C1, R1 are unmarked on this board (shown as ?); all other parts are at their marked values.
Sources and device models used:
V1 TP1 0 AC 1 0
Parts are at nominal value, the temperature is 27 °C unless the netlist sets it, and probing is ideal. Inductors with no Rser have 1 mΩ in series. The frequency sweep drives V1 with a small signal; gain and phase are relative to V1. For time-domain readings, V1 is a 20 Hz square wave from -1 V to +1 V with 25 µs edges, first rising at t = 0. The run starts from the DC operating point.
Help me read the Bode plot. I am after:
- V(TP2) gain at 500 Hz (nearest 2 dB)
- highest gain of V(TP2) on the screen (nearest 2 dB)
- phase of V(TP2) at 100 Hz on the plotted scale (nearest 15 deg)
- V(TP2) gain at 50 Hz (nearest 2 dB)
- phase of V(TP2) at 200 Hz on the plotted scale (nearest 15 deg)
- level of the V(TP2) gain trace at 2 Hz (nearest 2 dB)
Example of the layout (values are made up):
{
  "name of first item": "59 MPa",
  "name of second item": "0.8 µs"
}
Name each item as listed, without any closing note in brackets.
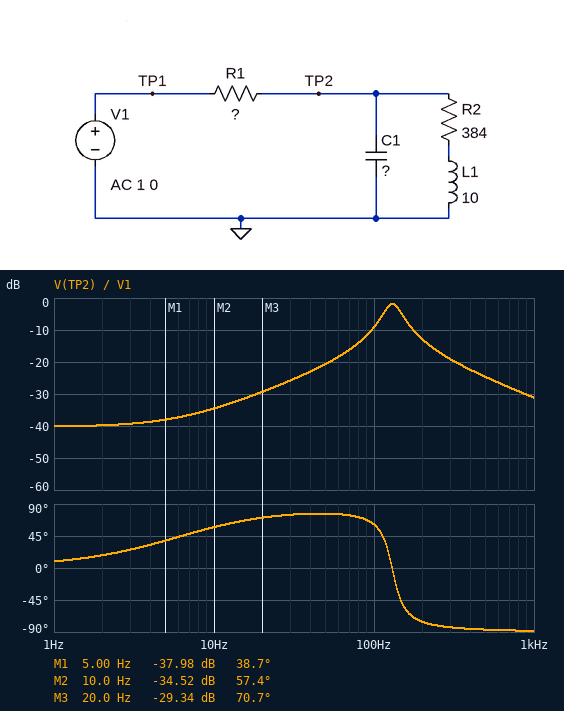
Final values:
{
  "V(TP2) gain at 500 Hz": "-24 dB",
  "highest gain of V(TP2) on the screen": "-2 dB",
  "phase of V(TP2) at 100 Hz on the plotted scale": "60 deg",
  "V(TP2) gain at 50 Hz": "-20 dB",
  "phase of V(TP2) at 200 Hz on the plotted scale": "-75 deg",
  "level of the V(TP2) gain trace at 2 Hz": "-40 dB"
}
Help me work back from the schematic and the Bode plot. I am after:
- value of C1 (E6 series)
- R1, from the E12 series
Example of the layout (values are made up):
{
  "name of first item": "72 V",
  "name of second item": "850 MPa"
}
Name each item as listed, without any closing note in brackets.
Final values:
{
  "value of C1": "150 nF",
  "R1, from the E12 series": "39 kΩ"
}
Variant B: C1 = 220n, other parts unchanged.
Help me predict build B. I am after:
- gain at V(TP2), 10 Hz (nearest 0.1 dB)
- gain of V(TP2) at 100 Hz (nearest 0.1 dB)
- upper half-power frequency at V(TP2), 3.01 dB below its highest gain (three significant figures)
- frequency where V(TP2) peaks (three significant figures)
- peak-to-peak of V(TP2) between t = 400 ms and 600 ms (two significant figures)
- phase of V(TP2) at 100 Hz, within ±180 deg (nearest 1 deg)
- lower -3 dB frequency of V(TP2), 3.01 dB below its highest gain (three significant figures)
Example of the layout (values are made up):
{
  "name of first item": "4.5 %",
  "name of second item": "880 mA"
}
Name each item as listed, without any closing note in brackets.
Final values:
{
  "gain at V(TP2), 10 Hz": "-34.5 dB",
  "gain of V(TP2) at 100 Hz": "-4.0 dB",
  "upper half-power frequency at V(TP2), 3.01 dB below its highest gain": "121 Hz",
  "frequency where V(TP2) peaks": "108 Hz",
  "peak-to-peak of V(TP2) between t = 400 ms and 600 ms": "640 mV",
  "phase of V(TP2) at 100 Hz, within ±180 deg": "30 deg",
  "lower -3 dB frequency of V(TP2), 3.01 dB below its highest gain": "96.2 Hz"
}
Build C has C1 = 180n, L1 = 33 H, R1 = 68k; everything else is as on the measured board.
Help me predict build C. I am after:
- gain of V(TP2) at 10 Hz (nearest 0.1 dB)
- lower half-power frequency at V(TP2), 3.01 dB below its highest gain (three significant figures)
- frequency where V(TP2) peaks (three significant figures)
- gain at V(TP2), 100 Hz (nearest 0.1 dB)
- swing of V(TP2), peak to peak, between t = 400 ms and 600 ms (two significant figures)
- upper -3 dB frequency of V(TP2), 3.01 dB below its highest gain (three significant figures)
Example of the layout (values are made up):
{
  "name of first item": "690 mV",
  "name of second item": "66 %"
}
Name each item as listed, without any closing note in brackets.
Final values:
{
  "gain of V(TP2) at 10 Hz": "-30.0 dB",
  "lower half-power frequency at V(TP2), 3.01 dB below its highest gain": "58.5 Hz",
  "frequency where V(TP2) peaks": "65.5 Hz",
  "gain at V(TP2), 100 Hz": "-13.1 dB",
  "swing of V(TP2), peak to peak, between t = 400 ms and 600 ms": "860 mV",
  "upper -3 dB frequency of V(TP2), 3.01 dB below its highest gain": "73.3 Hz"
}
